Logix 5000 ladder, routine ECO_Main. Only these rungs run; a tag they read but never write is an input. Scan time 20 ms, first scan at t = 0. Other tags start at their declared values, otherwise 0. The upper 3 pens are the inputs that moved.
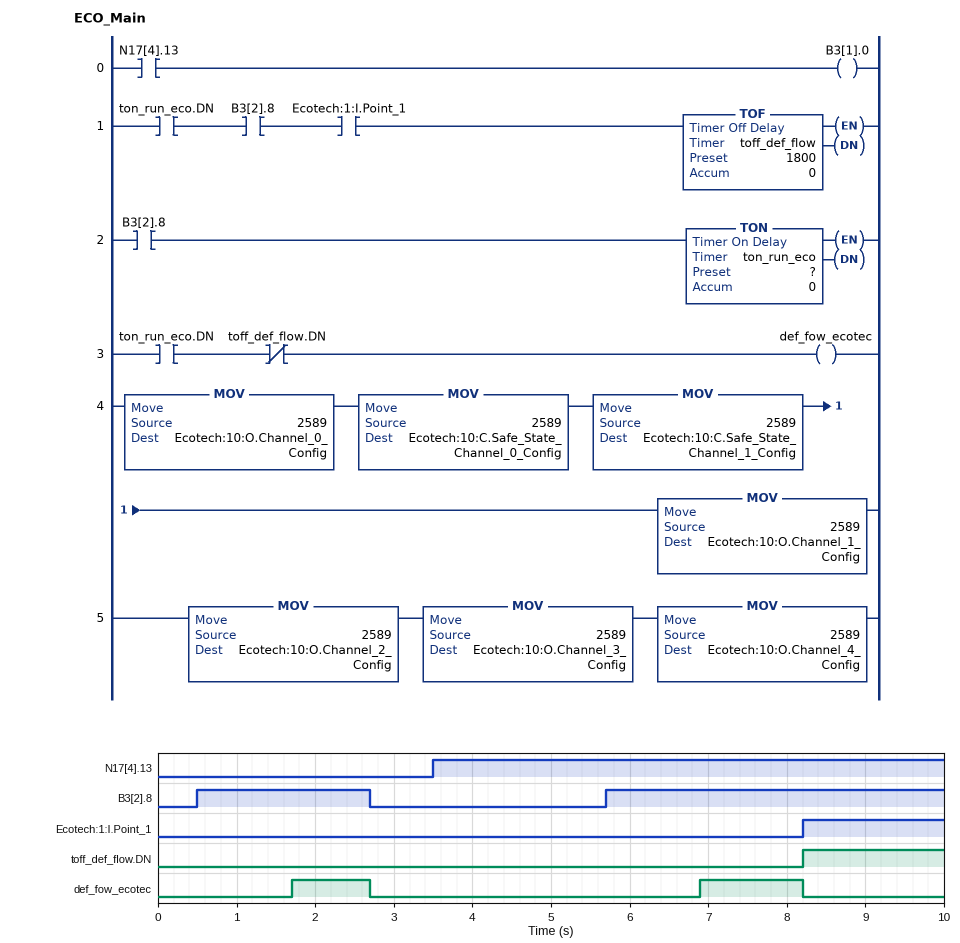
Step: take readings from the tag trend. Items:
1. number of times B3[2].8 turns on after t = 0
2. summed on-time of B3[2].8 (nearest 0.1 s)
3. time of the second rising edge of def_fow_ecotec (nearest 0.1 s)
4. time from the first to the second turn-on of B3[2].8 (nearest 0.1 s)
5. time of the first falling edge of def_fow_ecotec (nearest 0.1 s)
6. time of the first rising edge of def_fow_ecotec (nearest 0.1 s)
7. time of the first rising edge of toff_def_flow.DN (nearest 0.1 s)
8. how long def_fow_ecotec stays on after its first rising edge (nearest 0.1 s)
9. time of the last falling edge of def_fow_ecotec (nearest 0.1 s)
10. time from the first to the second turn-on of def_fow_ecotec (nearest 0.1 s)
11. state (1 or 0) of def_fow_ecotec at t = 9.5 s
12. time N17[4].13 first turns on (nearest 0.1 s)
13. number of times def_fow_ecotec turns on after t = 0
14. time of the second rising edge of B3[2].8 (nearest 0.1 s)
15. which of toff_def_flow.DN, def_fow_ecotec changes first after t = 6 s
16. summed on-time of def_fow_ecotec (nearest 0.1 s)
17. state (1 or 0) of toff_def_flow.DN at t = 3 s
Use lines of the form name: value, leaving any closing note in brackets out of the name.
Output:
number of times B3[2].8 turns on after t = 0: 2
summed on-time of B3[2].8: 6.5 s
time of the second rising edge of def_fow_ecotec: 6.9 s
time from the first to the second turn-on of B3[2].8: 5.2 s
time of the first falling edge of def_fow_ecotec: 2.7 s
time of the first rising edge of def_fow_ecotec: 1.7 s
time of the first rising edge of toff_def_flow.DN: 8.2 s
how long def_fow_ecotec stays on after its first rising edge: 1.0 s
time of the last falling edge of def_fow_ecotec: 8.2 s
time from the first to the second turn-on of def_fow_ecotec: 5.2 s
state (1 or 0) of def_fow_ecotec at t = 9.5 s: 0
time N17[4].13 first turns on: 3.5 s
number of times def_fow_ecotec turns on after t = 0: 2
time of the second rising edge of B3[2].8: 5.7 s
which of toff_def_flow.DN, def_fow_ecotec changes first after t = 6 s: def_fow_ecotec
summed on-time of def_fow_ecotec: 2.3 s
state (1 or 0) of toff_def_flow.DN at t = 3 s: 0
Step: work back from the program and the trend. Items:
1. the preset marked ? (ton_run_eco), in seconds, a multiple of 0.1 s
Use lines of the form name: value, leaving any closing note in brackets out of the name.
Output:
the preset marked ? (ton_run_eco), in seconds, a multiple of 0.1 s: 1.2 s
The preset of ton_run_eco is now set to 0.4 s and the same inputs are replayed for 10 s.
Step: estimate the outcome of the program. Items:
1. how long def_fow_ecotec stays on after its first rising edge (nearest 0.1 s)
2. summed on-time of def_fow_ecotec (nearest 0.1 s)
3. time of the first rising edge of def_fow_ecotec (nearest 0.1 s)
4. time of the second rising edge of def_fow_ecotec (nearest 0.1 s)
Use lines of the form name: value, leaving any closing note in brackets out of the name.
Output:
how long def_fow_ecotec stays on after its first rising edge: 1.8 s
summed on-time of def_fow_ecotec: 3.9 s
time of the first rising edge of def_fow_ecotec: 0.9 s
time of the second rising edge of def_fow_ecotec: 6.1 s
